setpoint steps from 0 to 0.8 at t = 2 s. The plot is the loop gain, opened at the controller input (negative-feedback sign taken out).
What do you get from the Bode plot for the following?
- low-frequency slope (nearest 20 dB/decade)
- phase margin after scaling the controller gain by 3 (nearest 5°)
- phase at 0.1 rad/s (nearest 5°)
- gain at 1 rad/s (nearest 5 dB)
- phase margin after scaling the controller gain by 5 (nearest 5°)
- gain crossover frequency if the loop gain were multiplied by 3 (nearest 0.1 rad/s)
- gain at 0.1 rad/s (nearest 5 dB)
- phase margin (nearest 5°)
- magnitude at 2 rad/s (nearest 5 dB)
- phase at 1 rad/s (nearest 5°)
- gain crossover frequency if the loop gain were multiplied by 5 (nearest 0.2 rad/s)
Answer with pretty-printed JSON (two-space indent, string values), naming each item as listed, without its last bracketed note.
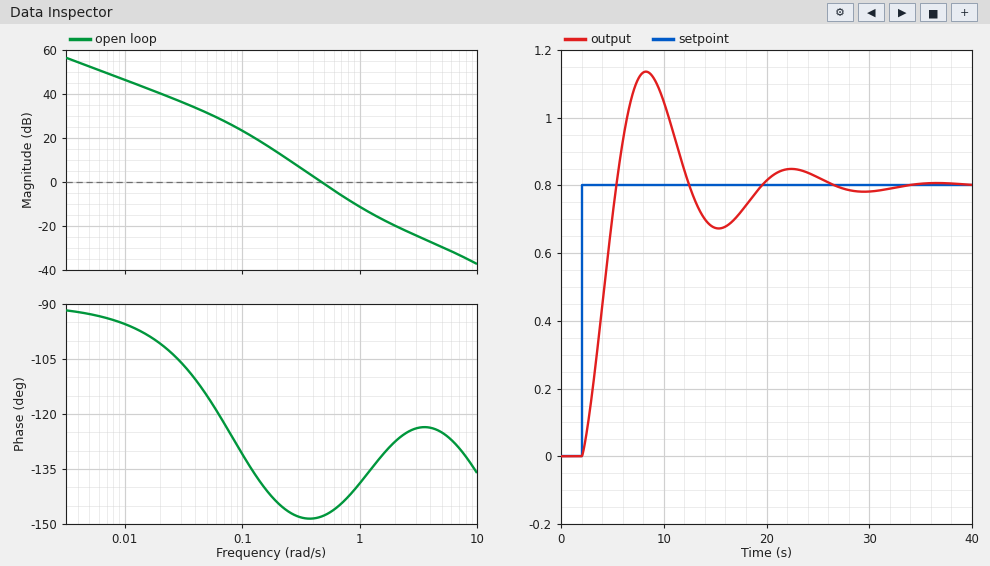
{
  "low-frequency slope": "-20 dB/decade",
  "phase margin after scaling the controller gain by 3": "40°",
  "phase at 0.1 rad/s": "-130°",
  "gain at 1 rad/s": "-10 dB",
  "phase margin after scaling the controller gain by 5": "45°",
  "gain crossover frequency if the loop gain were multiplied by 3": "0.9 rad/s",
  "gain at 0.1 rad/s": "25 dB",
  "phase margin": "30°",
  "magnitude at 2 rad/s": "-20 dB",
  "phase at 1 rad/s": "-140°",
  "gain crossover frequency if the loop gain were multiplied by 5": "1.2 rad/s"
}
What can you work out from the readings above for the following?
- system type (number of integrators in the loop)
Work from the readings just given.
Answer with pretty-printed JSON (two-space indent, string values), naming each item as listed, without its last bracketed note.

{
  "system type": "1"
}
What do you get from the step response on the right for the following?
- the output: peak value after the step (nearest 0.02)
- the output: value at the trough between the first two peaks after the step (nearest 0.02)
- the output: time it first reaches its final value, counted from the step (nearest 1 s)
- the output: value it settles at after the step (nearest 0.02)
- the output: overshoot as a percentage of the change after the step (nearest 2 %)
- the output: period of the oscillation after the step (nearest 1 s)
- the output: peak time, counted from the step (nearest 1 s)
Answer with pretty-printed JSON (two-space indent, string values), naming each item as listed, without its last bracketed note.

{
  "the output: peak value after the step": "1.14",
  "the output: value at the trough between the first two peaks after the step": "0.68",
  "the output: time it first reaches its final value, counted from the step": "3 s",
  "the output: value it settles at after the step": "0.80",
  "the output: overshoot as a percentage of the change after the step": "42 %",
  "the output: period of the oscillation after the step": "14 s",
  "the output: peak time, counted from the step": "6 s"
}
